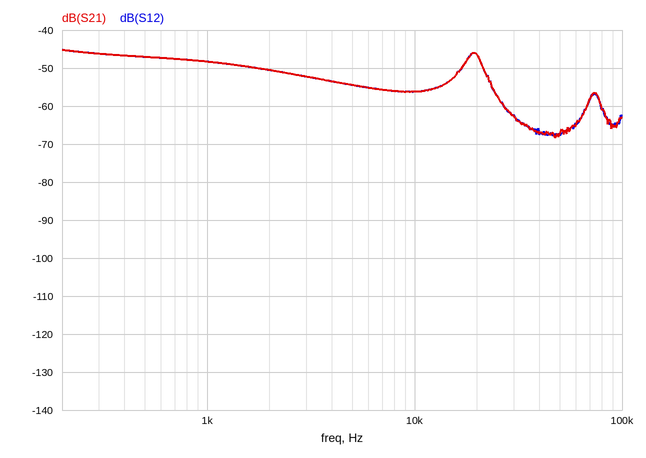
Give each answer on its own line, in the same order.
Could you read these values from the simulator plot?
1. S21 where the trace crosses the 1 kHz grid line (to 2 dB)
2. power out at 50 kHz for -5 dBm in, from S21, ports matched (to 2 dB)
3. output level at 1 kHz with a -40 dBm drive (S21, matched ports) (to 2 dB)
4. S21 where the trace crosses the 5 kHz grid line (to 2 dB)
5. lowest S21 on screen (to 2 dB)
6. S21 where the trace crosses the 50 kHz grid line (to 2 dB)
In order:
-48 dB
-72 dBm
-88 dBm
-54 dB
-68 dB
-68 dB
